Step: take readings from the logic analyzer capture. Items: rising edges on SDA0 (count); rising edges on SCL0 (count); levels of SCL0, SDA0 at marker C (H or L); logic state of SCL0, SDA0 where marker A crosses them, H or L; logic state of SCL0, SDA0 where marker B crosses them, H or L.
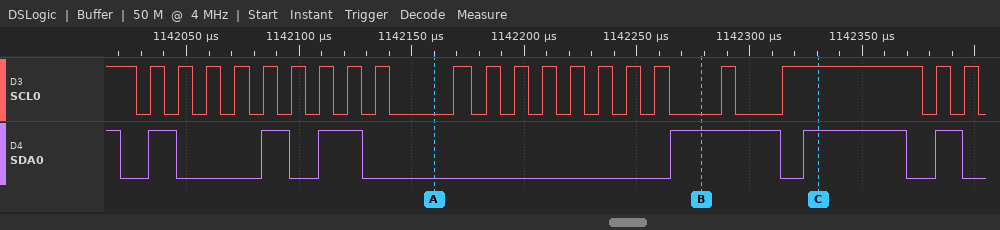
6
21
SCL0=H, SDA0=H
SCL0=L, SDA0=L
SCL0=L, SDA0=H
